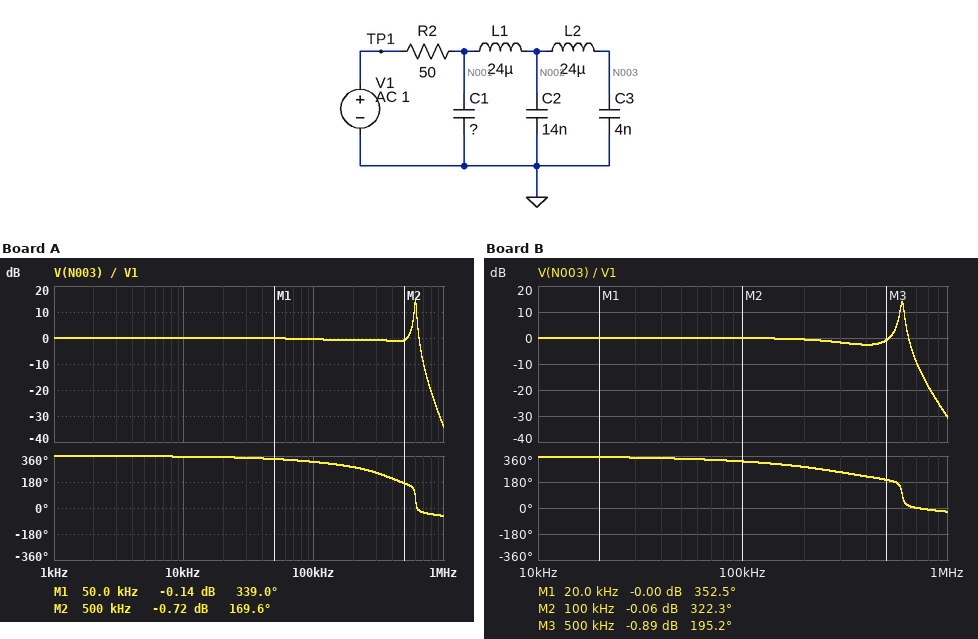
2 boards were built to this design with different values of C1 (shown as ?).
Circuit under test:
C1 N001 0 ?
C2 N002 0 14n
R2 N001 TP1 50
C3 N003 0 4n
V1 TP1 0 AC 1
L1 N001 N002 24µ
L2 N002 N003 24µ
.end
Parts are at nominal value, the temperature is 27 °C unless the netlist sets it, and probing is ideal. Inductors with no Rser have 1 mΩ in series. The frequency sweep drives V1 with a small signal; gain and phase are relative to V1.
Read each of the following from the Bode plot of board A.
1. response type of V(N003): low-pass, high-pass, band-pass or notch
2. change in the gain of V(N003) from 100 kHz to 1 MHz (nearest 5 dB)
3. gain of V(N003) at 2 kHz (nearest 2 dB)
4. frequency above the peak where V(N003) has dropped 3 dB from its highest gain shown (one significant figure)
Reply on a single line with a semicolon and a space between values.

low-pass; -35 dB; 0 dB; 600 kHz
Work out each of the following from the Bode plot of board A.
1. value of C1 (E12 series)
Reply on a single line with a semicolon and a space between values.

5.6 nF
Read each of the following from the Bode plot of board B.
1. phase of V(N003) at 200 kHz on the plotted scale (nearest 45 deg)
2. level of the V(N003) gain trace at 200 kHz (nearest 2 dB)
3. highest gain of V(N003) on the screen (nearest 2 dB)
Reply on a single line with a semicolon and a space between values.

270 deg; 0 dB; 14 dB
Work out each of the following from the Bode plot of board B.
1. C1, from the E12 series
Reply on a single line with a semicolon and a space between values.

2.7 nF
